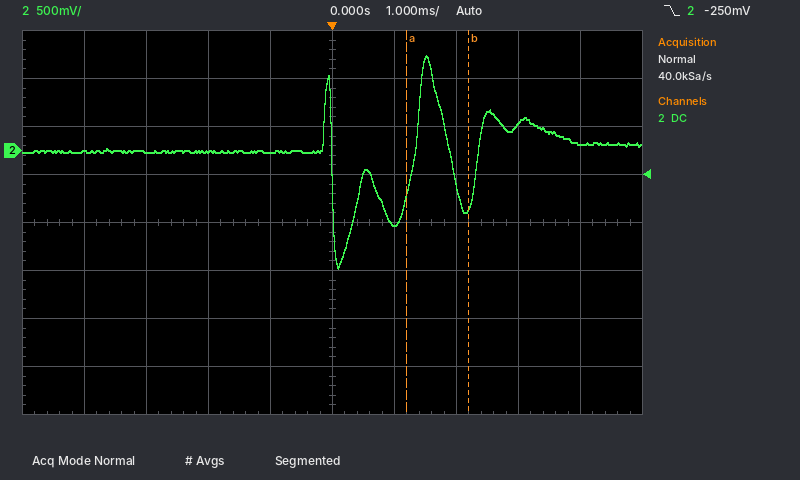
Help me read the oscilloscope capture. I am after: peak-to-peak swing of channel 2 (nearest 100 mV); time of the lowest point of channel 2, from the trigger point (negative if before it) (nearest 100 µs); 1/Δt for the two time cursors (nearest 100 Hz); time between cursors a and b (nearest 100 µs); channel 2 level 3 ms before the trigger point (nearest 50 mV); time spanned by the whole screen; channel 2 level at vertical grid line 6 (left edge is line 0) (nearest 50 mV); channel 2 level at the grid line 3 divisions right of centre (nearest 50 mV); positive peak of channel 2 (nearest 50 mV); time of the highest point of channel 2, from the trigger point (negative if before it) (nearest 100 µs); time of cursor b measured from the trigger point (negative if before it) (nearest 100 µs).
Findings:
2.20 V
+100 µs
1.0 kHz
1.0 ms
0 mV
10 ms
-750 mV
300 mV
1.00 V
+1.5 ms
+2.2 ms
